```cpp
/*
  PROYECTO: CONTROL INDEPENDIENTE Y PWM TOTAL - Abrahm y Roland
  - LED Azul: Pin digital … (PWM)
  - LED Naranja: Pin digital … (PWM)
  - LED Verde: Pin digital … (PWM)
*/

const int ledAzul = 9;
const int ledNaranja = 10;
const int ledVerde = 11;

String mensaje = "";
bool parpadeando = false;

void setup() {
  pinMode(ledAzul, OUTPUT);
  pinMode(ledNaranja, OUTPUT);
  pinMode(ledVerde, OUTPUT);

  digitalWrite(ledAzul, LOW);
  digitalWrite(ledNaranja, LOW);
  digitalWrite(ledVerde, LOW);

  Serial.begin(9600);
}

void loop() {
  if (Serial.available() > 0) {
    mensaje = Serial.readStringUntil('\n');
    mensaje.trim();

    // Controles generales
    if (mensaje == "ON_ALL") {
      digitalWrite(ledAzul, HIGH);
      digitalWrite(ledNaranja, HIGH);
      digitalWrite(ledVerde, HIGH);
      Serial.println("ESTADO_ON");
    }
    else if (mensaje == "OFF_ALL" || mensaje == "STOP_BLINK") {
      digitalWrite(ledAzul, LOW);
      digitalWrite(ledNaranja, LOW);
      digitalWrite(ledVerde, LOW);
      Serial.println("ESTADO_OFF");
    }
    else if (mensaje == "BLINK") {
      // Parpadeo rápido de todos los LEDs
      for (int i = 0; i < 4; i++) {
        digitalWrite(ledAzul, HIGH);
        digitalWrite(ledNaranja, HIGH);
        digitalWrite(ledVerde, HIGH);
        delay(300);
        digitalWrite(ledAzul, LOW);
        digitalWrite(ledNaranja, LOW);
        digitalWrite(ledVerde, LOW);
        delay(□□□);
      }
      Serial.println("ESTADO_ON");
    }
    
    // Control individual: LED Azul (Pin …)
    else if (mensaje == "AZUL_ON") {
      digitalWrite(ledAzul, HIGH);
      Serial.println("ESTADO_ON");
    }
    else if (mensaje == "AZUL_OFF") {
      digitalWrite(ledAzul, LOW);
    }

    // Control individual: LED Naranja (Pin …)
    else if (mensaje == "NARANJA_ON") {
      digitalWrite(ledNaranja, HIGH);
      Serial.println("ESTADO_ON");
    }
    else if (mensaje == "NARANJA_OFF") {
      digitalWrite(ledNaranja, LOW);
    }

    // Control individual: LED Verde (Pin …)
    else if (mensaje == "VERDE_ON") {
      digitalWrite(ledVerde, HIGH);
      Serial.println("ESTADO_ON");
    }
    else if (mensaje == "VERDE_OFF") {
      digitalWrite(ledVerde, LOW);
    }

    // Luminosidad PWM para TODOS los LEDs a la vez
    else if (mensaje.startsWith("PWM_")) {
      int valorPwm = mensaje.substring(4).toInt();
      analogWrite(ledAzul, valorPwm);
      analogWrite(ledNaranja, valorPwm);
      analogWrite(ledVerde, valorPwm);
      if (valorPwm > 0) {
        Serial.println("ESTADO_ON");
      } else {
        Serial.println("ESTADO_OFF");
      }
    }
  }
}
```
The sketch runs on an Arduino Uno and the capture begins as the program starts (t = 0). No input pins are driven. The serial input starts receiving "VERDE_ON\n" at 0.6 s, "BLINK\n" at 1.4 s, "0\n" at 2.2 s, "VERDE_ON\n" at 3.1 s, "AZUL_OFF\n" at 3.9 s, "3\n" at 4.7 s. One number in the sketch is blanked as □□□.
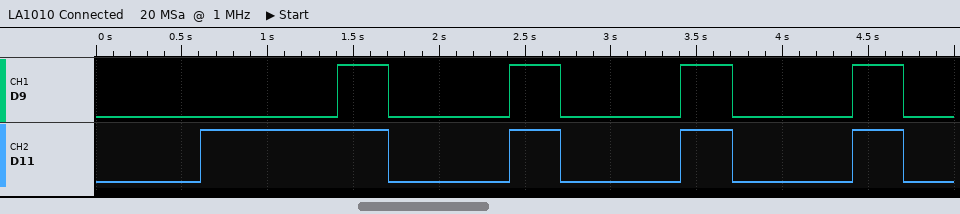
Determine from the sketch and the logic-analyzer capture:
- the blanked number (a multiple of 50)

700
